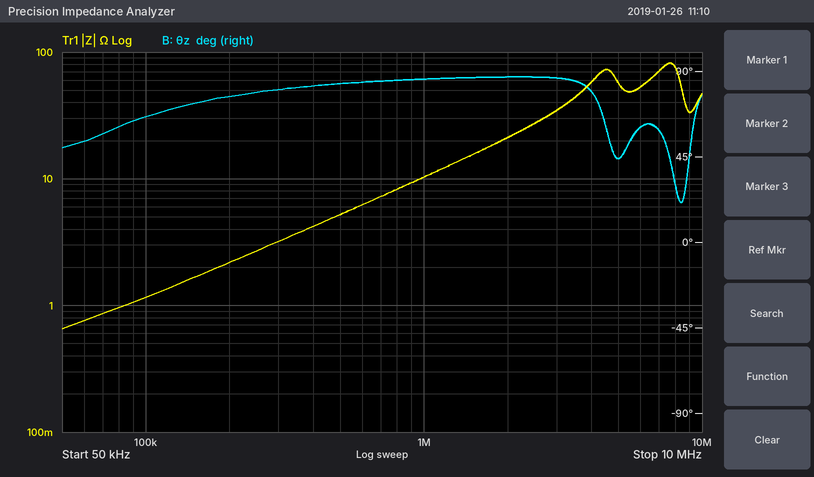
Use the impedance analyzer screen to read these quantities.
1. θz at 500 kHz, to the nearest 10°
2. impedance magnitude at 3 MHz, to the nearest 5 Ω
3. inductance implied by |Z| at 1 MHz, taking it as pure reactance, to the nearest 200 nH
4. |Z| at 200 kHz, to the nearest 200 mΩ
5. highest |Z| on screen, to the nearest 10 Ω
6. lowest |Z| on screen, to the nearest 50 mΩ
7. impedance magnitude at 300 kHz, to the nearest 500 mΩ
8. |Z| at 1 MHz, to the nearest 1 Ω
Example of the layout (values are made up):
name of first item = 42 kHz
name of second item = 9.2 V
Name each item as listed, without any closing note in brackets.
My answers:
θz at 500 kHz, to the nearest 10° = 80°
impedance magnitude at 3 MHz, to the nearest 5 Ω = 35 Ω
inductance implied by |Z| at 1 MHz, taking it as pure reactance, to the nearest 200 nH = 1.6 µH
|Z| at 200 kHz, to the nearest 200 mΩ = 2.2 Ω
highest |Z| on screen, to the nearest 10 Ω = 80 Ω
lowest |Z| on screen, to the nearest 50 mΩ = 650 mΩ
impedance magnitude at 300 kHz, to the nearest 500 mΩ = 3.0 Ω
|Z| at 1 MHz, to the nearest 1 Ω = 10 Ω
